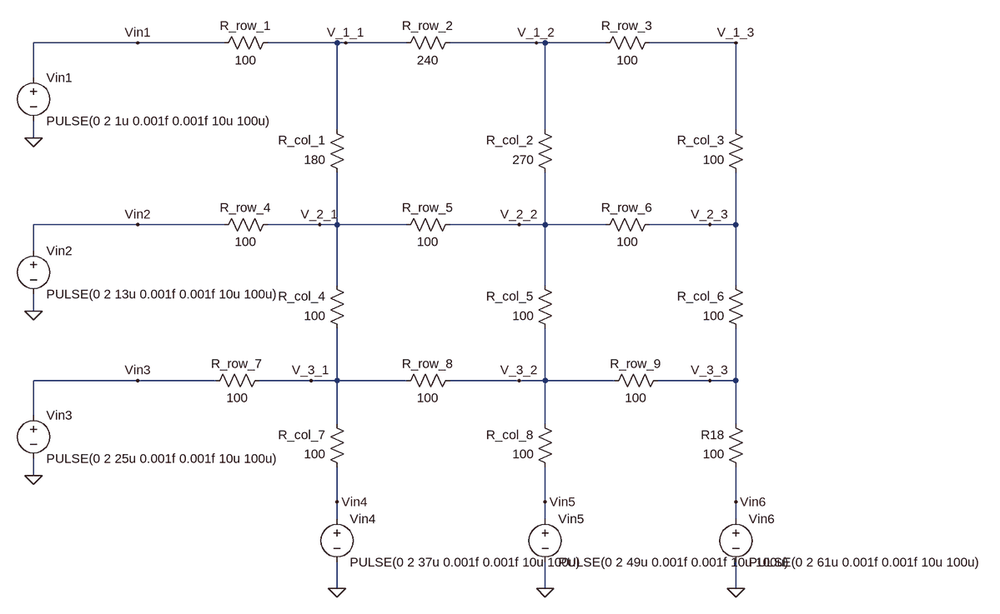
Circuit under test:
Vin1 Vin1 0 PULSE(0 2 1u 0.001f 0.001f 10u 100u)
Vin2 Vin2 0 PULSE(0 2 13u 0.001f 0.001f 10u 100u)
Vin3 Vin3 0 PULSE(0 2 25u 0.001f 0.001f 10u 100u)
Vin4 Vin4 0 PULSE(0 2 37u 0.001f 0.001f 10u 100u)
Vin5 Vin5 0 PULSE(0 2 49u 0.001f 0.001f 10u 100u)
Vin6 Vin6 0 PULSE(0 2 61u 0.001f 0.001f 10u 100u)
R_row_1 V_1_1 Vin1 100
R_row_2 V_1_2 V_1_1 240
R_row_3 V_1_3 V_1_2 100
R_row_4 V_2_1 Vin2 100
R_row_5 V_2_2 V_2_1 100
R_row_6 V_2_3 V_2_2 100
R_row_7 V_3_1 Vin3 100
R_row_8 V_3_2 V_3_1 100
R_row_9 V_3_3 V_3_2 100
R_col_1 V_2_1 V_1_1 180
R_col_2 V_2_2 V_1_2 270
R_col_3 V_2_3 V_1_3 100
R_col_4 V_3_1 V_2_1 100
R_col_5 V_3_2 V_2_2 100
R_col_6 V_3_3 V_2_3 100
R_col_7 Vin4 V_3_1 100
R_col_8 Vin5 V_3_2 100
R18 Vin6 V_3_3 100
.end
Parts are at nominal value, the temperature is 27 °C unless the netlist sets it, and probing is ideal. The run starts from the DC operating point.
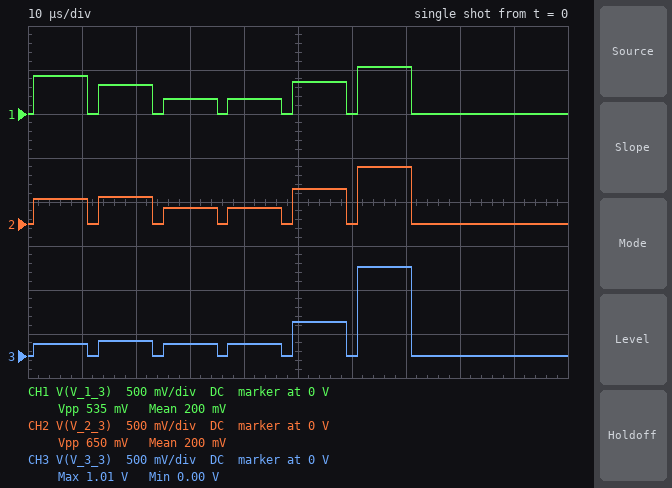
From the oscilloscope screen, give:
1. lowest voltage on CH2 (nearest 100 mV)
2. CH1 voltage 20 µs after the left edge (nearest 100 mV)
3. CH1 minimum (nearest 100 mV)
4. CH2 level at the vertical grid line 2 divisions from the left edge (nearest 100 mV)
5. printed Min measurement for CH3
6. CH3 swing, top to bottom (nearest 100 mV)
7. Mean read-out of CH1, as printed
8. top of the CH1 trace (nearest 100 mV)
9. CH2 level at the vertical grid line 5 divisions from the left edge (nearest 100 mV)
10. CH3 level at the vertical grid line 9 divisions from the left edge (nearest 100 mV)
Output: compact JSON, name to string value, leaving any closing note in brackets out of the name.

{"lowest voltage on CH2": "0 V", "CH1 voltage 20 µs after the left edge": "300 mV", "CH1 minimum": "0 V", "CH2 level at the vertical grid line 2 divisions from the left edge": "300 mV", "printed Min measurement for CH3": "0.00 V", "CH3 swing, top to bottom": "1.0 V", "Mean read-out of CH1, as printed": "200 mV", "top of the CH1 trace": "500 mV", "CH2 level at the vertical grid line 5 divisions from the left edge": "400 mV", "CH3 level at the vertical grid line 9 divisions from the left edge": "0 V"}
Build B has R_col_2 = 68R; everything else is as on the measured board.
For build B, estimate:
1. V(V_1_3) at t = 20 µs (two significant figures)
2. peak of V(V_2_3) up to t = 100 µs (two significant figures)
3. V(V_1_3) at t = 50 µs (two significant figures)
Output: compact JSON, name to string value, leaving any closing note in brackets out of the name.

{"V(V_1_3) at t = 20 µs": "350 mV", "peak of V(V_2_3) up to t = 100 µs": "650 mV", "V(V_1_3) at t = 50 µs": "390 mV"}
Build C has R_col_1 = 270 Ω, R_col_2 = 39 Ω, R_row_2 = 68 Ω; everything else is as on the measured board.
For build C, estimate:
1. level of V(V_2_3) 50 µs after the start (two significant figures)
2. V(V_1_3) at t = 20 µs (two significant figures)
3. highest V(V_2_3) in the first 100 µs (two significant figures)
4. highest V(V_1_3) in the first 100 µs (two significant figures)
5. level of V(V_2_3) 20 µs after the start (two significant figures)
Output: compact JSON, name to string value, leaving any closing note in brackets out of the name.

{"level of V(V_2_3) 50 µs after the start": "370 mV", "V(V_1_3) at t = 20 µs": "330 mV", "highest V(V_2_3) in the first 100 µs": "610 mV", "highest V(V_1_3) in the first 100 µs": "520 mV", "level of V(V_2_3) 20 µs after the start": "300 mV"}
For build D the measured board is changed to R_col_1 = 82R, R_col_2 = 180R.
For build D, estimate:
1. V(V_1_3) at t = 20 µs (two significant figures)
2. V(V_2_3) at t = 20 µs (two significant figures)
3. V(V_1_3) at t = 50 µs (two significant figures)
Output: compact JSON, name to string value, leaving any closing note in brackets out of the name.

{"V(V_1_3) at t = 20 µs": "340 mV", "V(V_2_3) at t = 20 µs": "310 mV", "V(V_1_3) at t = 50 µs": "370 mV"}
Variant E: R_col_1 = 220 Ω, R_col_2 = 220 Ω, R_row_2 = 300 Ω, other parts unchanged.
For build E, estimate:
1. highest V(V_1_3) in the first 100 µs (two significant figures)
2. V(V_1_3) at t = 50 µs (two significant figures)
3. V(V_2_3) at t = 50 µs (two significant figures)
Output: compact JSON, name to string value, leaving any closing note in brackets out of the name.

{"highest V(V_1_3) in the first 100 µs": "550 mV", "V(V_1_3) at t = 50 µs": "380 mV", "V(V_2_3) at t = 50 µs": "410 mV"}
